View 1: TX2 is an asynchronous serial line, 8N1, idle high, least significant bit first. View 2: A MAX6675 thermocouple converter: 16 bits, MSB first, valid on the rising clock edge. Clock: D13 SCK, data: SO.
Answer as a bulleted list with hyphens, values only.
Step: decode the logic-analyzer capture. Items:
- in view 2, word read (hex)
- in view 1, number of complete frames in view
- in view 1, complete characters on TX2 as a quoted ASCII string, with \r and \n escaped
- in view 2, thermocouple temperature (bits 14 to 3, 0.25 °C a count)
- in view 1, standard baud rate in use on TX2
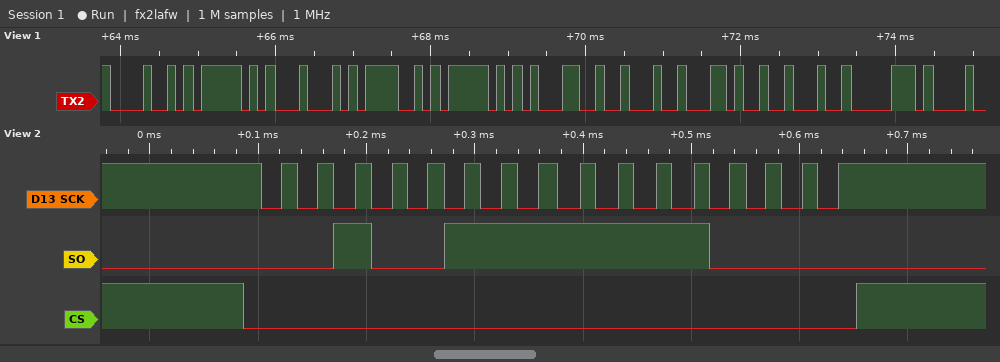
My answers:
- 0x27F0
- 10
- "H_DO_1\",\"p"
- 319.50 °C
- 9600 baud
